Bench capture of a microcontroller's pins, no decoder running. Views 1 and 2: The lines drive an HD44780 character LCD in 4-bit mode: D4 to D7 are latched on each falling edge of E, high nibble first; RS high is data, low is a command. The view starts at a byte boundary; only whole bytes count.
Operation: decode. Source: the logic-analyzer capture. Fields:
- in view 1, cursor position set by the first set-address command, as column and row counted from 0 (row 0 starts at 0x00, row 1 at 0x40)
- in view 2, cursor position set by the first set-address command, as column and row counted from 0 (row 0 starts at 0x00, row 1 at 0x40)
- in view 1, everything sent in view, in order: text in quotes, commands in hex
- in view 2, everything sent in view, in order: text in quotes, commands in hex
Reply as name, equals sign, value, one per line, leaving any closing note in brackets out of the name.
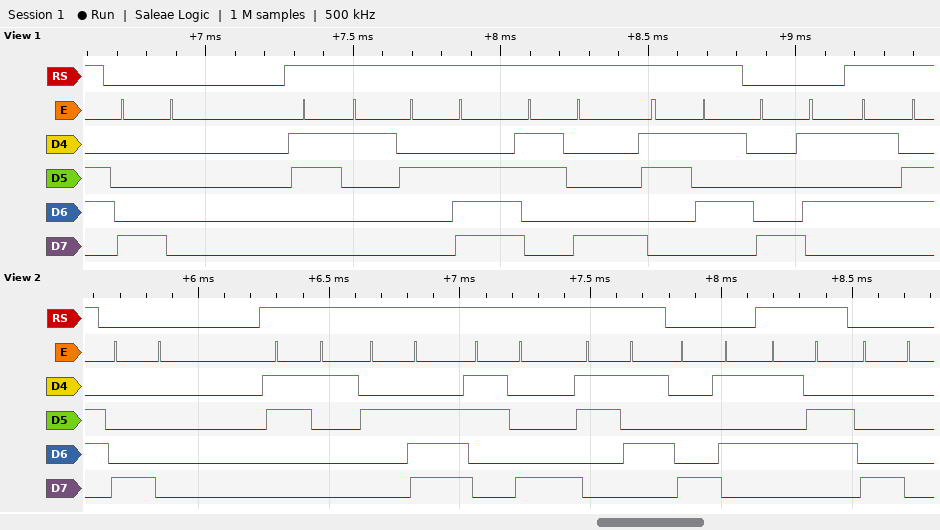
in view 1, cursor position set by the first set-address command, as column and row counted from 0 = column 0, row 0
in view 2, cursor position set by the first set-address command, as column and row counted from 0 = column 0, row 0
in view 1, everything sent in view, in order: text in quotes, commands in hex = 0x80 "1.85" 0x85 "V"
in view 2, everything sent in view, in order: text in quotes, commands in hex = 0x80 "1.85" 0x85 "V" 0x80
